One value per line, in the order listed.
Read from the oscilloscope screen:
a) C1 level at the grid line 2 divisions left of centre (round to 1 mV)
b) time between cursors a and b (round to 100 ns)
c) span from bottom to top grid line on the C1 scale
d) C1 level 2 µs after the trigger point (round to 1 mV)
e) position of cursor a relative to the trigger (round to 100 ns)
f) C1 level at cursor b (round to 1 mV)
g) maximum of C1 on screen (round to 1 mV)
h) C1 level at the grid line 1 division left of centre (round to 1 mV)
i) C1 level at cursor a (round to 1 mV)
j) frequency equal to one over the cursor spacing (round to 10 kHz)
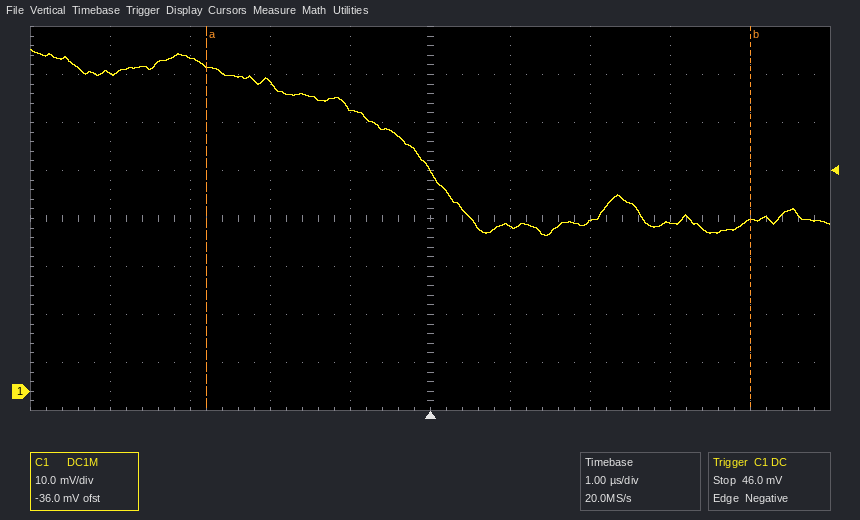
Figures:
64 mV
6.8 µs
80 mV
35 mV
-2.8 µs
36 mV
71 mV
59 mV
68 mV
150 kHz
